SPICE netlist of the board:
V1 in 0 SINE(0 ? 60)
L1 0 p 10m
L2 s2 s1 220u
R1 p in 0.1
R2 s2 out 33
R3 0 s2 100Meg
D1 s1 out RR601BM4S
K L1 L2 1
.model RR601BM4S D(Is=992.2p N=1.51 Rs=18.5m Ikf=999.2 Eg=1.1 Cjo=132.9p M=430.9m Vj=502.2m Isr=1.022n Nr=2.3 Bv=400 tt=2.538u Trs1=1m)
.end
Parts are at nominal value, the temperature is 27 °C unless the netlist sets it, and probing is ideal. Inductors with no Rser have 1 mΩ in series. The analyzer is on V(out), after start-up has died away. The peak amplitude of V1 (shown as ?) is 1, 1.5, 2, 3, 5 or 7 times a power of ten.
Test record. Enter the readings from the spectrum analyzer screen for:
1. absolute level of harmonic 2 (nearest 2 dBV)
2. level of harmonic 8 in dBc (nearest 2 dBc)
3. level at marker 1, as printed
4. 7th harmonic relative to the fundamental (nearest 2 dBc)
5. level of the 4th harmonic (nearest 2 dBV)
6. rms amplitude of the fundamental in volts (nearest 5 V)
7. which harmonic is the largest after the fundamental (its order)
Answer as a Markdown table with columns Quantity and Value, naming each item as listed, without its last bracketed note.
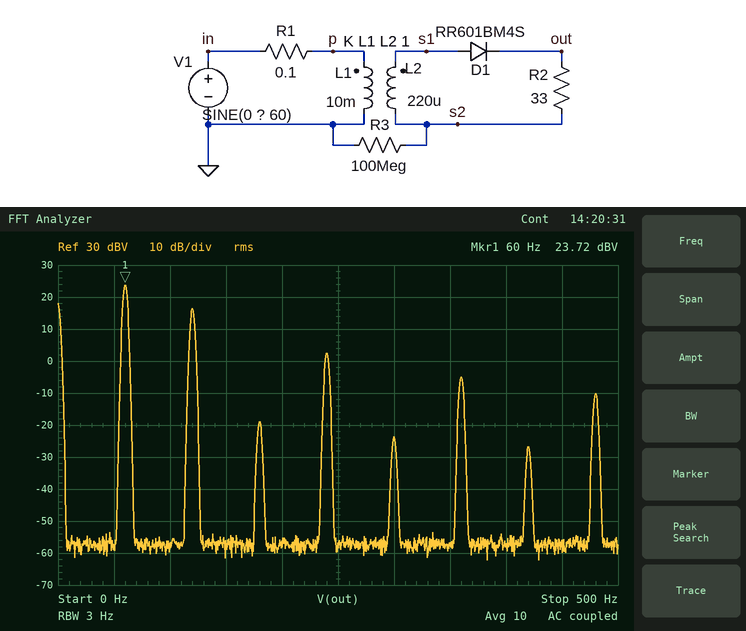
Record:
| Quantity | Value |
|---|---|
| absolute level of harmonic 2 | 16 dBV |
| level of harmonic 8 in dBc | -34 dBc |
| level at marker 1, as printed | 23.72 dBV |
| 7th harmonic relative to the fundamental | -50 dBc |
| level of the 4th harmonic | 2 dBV |
| rms amplitude of the fundamental in volts | 15 V |
| which harmonic is the largest after the fundamental | 2 |
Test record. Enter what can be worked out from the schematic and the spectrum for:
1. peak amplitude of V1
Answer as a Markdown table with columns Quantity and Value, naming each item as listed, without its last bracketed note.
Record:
| Quantity | Value |
|---|---|
| peak amplitude of V1 | 300 V |
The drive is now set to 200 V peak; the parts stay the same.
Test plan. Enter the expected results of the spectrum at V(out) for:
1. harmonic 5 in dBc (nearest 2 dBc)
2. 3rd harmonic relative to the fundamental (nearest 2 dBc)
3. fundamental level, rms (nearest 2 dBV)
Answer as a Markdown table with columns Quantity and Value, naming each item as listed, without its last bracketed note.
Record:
| Quantity | Value |
|---|---|
| harmonic 5 in dBc | -44 dBc |
| 3rd harmonic relative to the fundamental | -40 dBc |
| fundamental level, rms | 20 dBV |
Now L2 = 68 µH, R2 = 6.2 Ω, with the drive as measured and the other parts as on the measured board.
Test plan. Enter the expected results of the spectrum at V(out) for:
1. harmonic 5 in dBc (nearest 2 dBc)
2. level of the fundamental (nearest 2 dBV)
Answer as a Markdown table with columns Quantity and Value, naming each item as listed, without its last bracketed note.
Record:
| Quantity | Value |
|---|---|
| harmonic 5 in dBc | -42 dBc |
| level of the fundamental | 18 dBV |
